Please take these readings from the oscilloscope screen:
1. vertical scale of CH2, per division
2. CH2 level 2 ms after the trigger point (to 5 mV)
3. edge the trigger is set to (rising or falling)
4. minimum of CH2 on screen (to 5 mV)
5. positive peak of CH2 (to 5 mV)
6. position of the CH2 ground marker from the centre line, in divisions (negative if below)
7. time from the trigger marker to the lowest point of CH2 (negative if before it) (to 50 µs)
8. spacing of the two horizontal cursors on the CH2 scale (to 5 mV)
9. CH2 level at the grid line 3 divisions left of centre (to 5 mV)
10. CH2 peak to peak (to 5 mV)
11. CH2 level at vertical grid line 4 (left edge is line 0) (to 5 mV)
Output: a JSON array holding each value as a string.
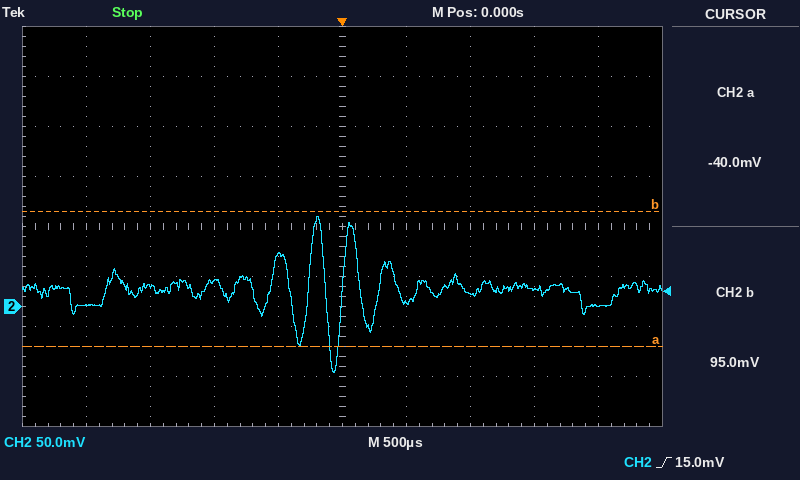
["50 mV", "0 mV", "rising", "-65 mV", "90 mV", "-1.6 div", "-50 µs", "135 mV", "20 mV", "155 mV", "50 mV"]
